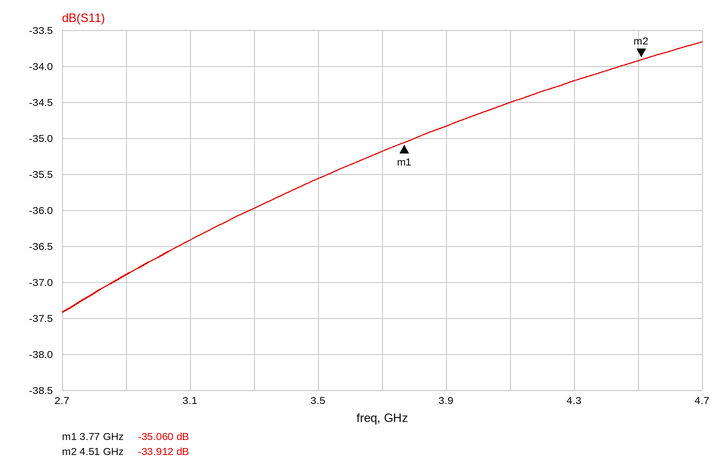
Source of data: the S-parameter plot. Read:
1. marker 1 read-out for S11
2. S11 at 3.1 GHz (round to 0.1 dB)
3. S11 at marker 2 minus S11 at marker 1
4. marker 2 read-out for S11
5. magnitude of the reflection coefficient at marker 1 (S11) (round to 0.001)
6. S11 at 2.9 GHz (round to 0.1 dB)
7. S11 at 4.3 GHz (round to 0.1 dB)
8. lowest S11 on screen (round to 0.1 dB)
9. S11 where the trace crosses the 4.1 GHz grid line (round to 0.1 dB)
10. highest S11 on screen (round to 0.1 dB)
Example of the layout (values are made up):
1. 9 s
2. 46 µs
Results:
1. -35.060 dB
2. -36.4 dB
3. 1.148 dB
4. -33.912 dB
5. 0.018
6. -36.9 dB
7. -34.2 dB
8. -37.4 dB
9. -34.5 dB
10. -33.7 dB
